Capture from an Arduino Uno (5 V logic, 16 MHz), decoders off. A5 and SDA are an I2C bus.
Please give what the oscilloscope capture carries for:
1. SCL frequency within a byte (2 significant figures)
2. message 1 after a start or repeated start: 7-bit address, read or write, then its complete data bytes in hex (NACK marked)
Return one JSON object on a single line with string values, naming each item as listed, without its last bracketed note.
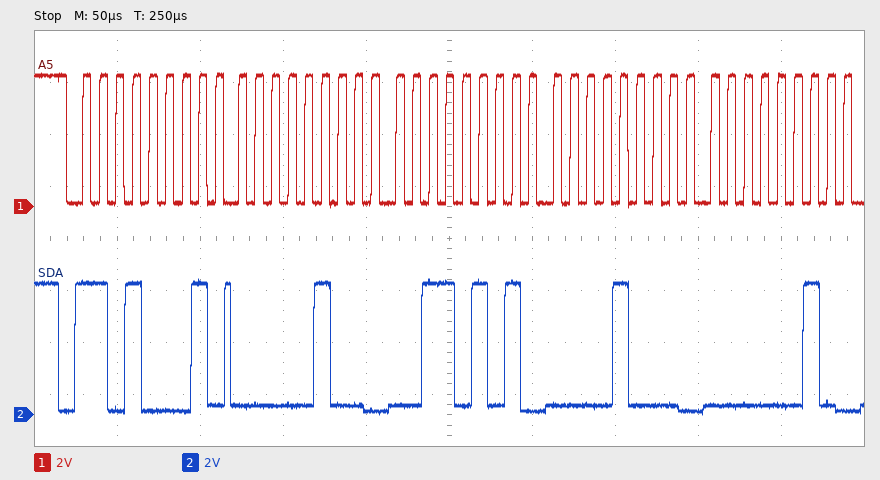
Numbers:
{"SCL frequency within a byte": "100 kHz", "message 1 after a start or repeated start: 7-bit address, read or write, then its complete data bytes in hex": "0x68 read: 04 35 08 02"}
